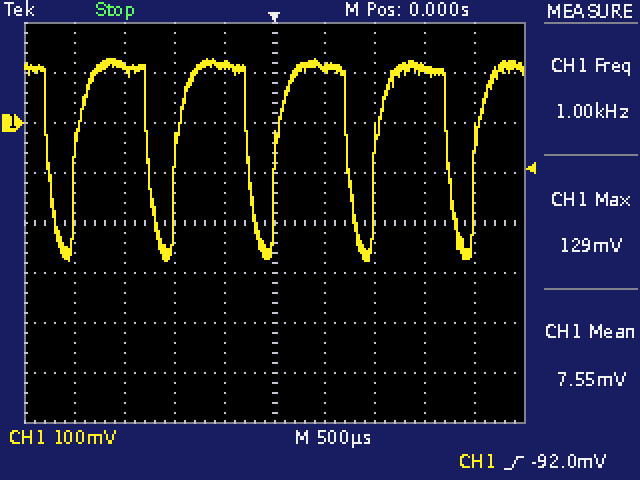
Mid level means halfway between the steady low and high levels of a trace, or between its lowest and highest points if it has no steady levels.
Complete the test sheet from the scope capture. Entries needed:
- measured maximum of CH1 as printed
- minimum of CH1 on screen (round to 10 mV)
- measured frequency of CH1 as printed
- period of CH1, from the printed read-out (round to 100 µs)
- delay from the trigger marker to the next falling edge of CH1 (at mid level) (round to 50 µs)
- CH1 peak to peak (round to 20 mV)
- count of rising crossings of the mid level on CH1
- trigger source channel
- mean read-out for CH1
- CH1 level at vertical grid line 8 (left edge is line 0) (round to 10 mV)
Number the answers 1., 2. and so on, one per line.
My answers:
1. 129 mV
2. -280 mV
3. 1.00 kHz
4. 1.0 ms
5. 750 µs
6. 400 mV
7. 5
8. CH1
9. 7.55 mV
10. 110 mV
